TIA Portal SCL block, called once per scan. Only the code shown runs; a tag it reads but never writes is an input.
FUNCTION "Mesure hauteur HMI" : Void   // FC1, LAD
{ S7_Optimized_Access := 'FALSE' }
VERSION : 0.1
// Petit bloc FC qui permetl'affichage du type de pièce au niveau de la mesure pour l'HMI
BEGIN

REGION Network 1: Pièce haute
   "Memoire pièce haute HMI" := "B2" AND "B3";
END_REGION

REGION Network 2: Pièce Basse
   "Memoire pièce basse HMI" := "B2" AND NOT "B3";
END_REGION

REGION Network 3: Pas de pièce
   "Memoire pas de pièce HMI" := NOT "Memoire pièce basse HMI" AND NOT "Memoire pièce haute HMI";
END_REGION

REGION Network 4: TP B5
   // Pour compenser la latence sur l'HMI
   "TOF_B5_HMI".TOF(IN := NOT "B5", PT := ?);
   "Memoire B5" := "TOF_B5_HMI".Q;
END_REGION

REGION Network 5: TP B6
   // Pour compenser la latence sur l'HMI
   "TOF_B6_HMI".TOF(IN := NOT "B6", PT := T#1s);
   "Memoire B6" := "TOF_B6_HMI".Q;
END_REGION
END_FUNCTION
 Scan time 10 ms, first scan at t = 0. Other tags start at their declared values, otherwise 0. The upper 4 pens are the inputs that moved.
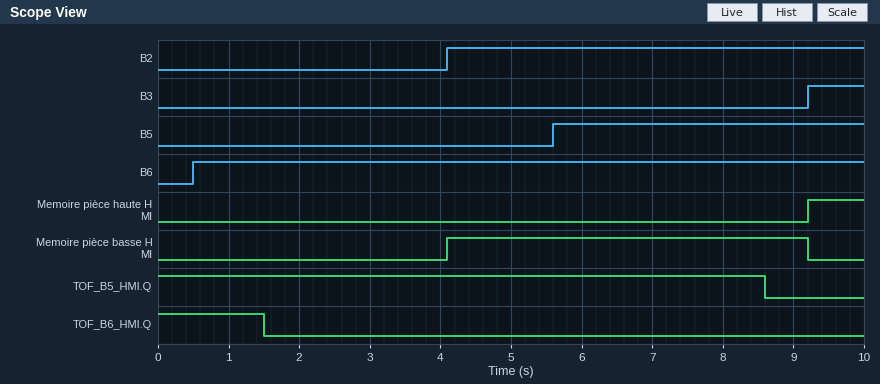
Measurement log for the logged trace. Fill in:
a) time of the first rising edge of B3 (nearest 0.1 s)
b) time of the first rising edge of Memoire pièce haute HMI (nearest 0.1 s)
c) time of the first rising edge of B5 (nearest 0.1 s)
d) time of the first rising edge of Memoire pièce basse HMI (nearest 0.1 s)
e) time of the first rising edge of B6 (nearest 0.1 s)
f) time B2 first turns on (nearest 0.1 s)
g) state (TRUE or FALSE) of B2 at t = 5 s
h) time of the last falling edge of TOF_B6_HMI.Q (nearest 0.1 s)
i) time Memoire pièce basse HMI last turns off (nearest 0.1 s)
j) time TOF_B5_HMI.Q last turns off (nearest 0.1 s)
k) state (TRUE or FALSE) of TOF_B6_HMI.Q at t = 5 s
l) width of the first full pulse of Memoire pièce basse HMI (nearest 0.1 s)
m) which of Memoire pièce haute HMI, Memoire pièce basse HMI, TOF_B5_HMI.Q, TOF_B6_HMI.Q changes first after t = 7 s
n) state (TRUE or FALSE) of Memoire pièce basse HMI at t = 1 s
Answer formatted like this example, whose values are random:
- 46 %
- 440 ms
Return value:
- 9.2 s
- 9.2 s
- 5.6 s
- 4.1 s
- 0.5 s
- 4.1 s
- TRUE
- 1.5 s
- 9.2 s
- 8.6 s
- FALSE
- 5.1 s
- TOF_B5_HMI.Q
- FALSE
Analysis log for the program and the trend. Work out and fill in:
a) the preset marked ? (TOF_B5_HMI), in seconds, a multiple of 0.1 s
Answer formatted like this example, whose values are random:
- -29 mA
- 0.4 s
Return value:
- 3.0 s
